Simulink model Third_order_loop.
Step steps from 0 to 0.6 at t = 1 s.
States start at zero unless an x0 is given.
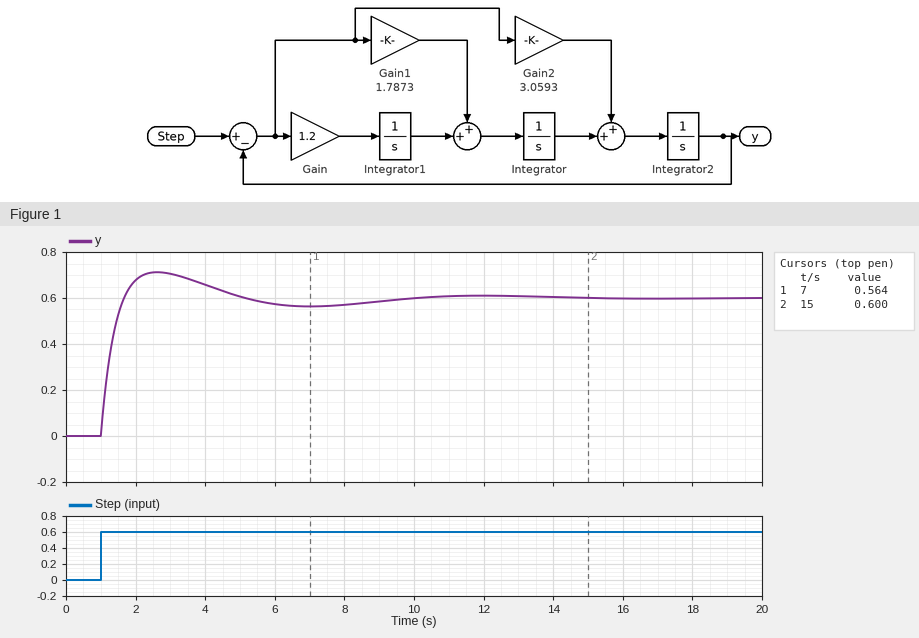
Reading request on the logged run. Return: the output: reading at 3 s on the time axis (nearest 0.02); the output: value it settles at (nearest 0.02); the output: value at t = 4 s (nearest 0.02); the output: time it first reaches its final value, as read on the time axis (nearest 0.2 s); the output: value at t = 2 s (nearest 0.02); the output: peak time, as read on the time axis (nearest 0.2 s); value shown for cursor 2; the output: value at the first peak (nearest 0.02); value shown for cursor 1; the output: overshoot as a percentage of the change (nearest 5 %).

0.70
0.60
0.66
1.6 s
0.68
2.6 s
0.600
0.72
0.564
20 %
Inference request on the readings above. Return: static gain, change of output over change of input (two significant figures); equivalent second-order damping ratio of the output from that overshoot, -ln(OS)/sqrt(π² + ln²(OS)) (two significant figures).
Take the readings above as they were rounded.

1.0
0.46
